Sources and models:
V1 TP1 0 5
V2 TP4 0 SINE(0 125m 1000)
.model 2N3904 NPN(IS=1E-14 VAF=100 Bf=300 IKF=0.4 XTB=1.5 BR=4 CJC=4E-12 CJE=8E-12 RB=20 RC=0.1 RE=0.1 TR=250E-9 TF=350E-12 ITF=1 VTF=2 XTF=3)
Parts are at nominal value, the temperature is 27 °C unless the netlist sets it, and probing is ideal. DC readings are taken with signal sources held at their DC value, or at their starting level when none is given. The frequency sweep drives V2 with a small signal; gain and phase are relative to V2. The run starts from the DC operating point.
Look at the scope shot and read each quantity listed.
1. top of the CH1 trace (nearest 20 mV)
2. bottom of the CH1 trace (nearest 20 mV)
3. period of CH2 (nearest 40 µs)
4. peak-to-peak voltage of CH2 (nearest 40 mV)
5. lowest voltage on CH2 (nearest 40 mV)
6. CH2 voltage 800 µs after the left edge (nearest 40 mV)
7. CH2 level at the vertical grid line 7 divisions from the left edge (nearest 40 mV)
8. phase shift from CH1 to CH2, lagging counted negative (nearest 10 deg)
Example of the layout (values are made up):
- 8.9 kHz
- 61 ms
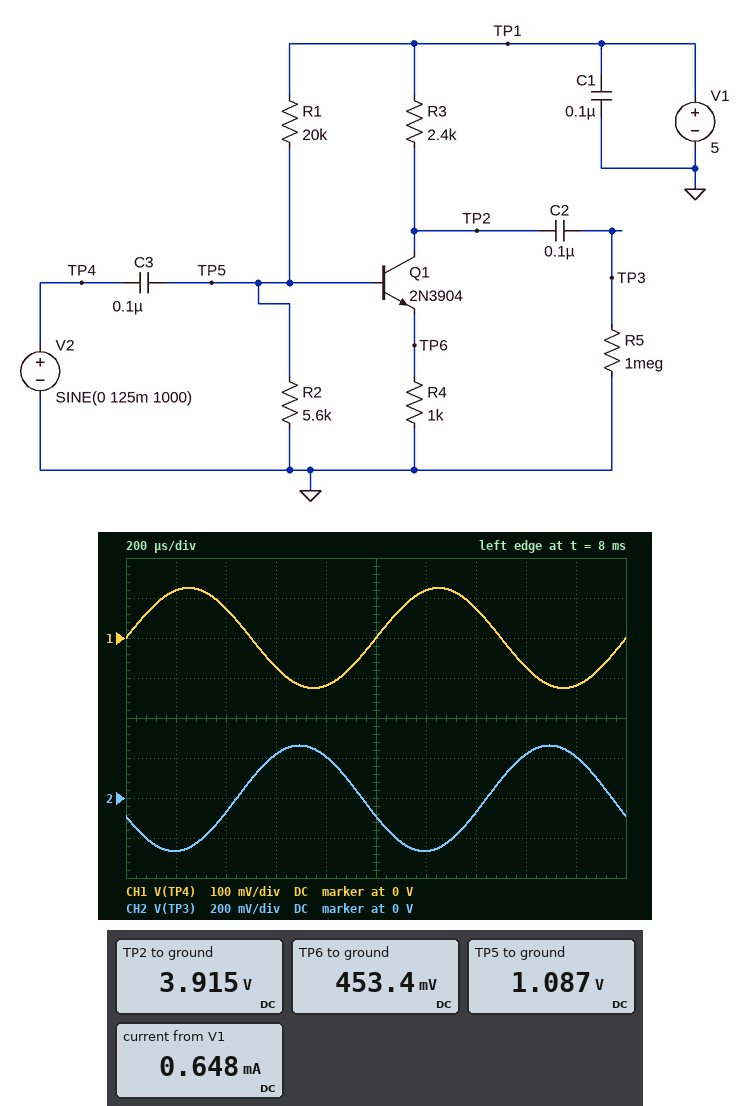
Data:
- 120 mV
- -120 mV
- 1.00 ms
- 520 mV
- -280 mV
- 200 mV
- -80 mV
- -160 deg
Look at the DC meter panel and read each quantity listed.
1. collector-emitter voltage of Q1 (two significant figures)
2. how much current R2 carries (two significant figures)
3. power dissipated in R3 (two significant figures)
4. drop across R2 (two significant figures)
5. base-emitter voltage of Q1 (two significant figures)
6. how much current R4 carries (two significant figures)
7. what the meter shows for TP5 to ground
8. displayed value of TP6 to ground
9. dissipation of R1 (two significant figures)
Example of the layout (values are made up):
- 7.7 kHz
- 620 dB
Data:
- 3.5 V
- 190 µA
- 490 µW
- 1.1 V
- 630 mV
- 450 µA
- 1.087 V
- 453.4 mV
- 770 µW
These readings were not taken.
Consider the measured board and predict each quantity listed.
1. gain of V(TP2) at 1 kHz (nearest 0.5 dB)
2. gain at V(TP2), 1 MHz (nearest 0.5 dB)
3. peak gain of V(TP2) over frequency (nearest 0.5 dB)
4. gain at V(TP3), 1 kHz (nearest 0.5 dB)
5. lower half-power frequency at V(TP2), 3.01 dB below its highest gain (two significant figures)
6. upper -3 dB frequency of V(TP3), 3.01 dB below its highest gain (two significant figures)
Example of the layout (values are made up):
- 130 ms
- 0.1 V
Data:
- 6.5 dB
- 7.0 dB
- 7.0 dB
- 6.5 dB
- 370 Hz
- 42 MHz
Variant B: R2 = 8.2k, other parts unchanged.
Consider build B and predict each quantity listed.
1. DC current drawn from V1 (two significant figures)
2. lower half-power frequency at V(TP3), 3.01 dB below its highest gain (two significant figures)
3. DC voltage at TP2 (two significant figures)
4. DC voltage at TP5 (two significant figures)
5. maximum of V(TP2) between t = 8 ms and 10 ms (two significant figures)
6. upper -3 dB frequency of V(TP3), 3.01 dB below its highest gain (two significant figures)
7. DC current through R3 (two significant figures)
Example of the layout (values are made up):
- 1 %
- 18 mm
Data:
- 970 µA
- 280 Hz
- 3.1 V
- 1.4 V
- 3.4 V
- 34 MHz
- 790 µA
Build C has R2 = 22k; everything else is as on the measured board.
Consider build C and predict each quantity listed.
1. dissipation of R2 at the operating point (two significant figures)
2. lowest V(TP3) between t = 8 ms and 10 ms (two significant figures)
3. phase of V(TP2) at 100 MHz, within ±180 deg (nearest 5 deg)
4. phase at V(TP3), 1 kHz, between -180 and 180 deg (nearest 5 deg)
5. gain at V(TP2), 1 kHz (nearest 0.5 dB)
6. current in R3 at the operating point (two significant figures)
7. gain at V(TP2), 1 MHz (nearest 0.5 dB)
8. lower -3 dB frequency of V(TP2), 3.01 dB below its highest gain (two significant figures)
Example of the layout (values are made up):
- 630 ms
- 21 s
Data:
- 210 µW
- -5.9 mV
- 0 deg
- 60 deg
- -16.5 dB
- 1.4 mA
- -0.5 dB
- 190 kHz
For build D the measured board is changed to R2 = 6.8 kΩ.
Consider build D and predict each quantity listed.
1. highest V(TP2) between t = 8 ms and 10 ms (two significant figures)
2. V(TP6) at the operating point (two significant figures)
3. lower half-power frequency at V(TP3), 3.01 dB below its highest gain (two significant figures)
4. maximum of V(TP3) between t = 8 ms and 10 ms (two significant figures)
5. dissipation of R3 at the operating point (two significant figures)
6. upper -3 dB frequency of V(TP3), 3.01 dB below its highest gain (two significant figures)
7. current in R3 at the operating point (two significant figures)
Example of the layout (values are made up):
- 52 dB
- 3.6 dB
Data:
- 3.8 V
- 620 mV
- 320 Hz
- 270 mV
- 910 µW
- 38 MHz
- 610 µA
